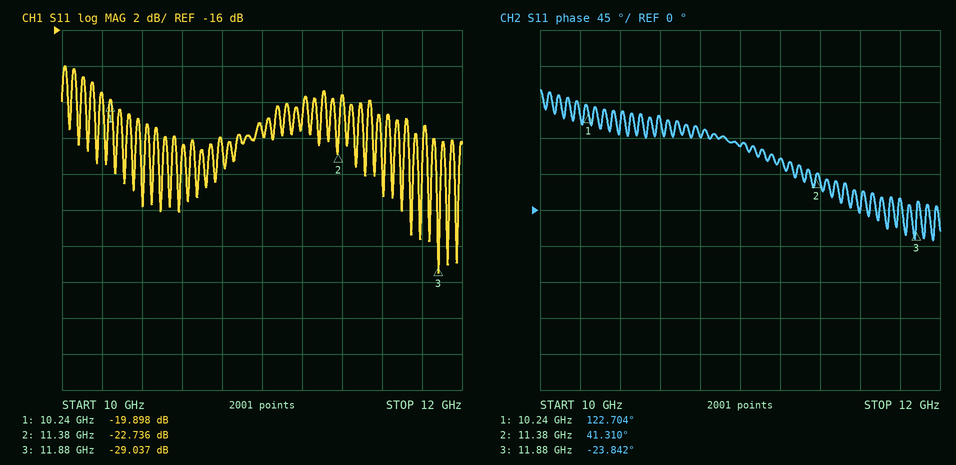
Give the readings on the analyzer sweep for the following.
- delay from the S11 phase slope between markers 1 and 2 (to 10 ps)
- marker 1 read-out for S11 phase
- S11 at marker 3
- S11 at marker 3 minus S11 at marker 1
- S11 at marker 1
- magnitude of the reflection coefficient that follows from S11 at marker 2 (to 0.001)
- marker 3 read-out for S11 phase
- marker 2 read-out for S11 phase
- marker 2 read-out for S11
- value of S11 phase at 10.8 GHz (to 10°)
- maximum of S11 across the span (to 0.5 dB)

200 ps
122.704°
-29.037 dB
-9.139 dB
-19.898 dB
0.073
-23.842°
41.310°
-22.736 dB
90°
-18.0 dB
